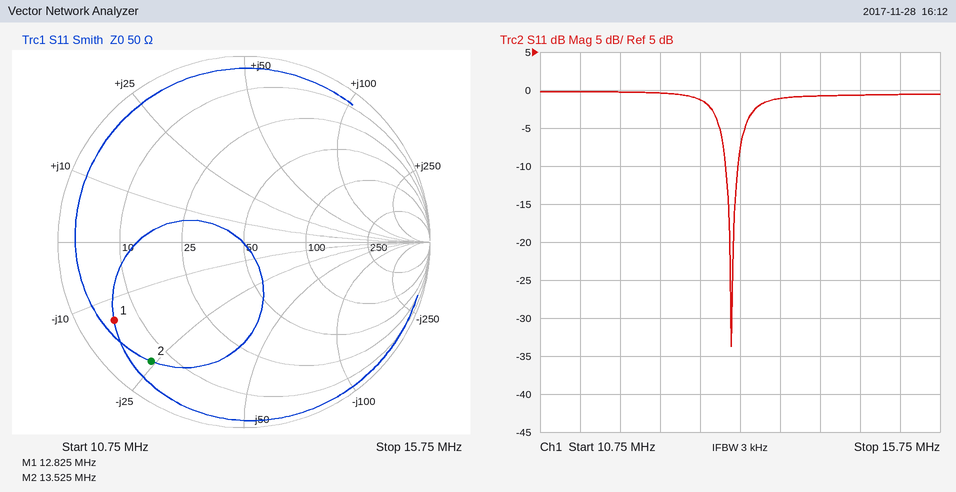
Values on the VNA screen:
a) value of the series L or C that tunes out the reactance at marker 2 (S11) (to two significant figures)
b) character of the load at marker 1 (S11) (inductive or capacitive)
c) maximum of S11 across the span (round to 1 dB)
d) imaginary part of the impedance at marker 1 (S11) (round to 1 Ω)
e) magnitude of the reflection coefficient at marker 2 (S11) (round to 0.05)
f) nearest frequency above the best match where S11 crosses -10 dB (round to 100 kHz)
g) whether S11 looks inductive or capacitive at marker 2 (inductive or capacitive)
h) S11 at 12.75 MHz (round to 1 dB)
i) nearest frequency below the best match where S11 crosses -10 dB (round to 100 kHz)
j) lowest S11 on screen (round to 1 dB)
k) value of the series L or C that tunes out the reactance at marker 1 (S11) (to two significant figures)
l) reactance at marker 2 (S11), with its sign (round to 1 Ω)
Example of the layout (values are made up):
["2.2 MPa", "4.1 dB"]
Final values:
["280 nH", "capacitive", "0 dB", "-14 Ω", "0.80", "13.2 MHz", "capacitive", "-1 dB", "13.1 MHz", "-34 dB", "170 nH", "-24 Ω"]
